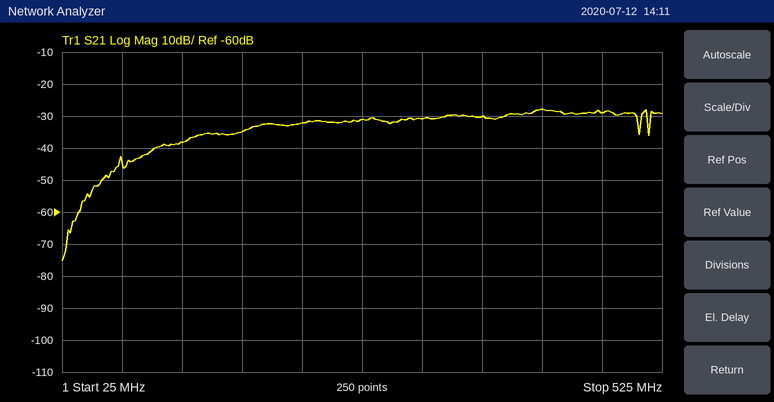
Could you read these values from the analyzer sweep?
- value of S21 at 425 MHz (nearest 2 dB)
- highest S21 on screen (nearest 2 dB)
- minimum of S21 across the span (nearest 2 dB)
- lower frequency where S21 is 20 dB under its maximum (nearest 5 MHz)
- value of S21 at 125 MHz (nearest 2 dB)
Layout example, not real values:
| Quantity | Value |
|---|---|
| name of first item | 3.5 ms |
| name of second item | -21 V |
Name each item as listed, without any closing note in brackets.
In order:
| Quantity | Value |
|---|---|
| value of S21 at 425 MHz | -28 dB |
| highest S21 on screen | -28 dB |
| minimum of S21 across the span | -76 dB |
| lower frequency where S21 is 20 dB under its maximum | 65 MHz |
| value of S21 at 125 MHz | -38 dB |
